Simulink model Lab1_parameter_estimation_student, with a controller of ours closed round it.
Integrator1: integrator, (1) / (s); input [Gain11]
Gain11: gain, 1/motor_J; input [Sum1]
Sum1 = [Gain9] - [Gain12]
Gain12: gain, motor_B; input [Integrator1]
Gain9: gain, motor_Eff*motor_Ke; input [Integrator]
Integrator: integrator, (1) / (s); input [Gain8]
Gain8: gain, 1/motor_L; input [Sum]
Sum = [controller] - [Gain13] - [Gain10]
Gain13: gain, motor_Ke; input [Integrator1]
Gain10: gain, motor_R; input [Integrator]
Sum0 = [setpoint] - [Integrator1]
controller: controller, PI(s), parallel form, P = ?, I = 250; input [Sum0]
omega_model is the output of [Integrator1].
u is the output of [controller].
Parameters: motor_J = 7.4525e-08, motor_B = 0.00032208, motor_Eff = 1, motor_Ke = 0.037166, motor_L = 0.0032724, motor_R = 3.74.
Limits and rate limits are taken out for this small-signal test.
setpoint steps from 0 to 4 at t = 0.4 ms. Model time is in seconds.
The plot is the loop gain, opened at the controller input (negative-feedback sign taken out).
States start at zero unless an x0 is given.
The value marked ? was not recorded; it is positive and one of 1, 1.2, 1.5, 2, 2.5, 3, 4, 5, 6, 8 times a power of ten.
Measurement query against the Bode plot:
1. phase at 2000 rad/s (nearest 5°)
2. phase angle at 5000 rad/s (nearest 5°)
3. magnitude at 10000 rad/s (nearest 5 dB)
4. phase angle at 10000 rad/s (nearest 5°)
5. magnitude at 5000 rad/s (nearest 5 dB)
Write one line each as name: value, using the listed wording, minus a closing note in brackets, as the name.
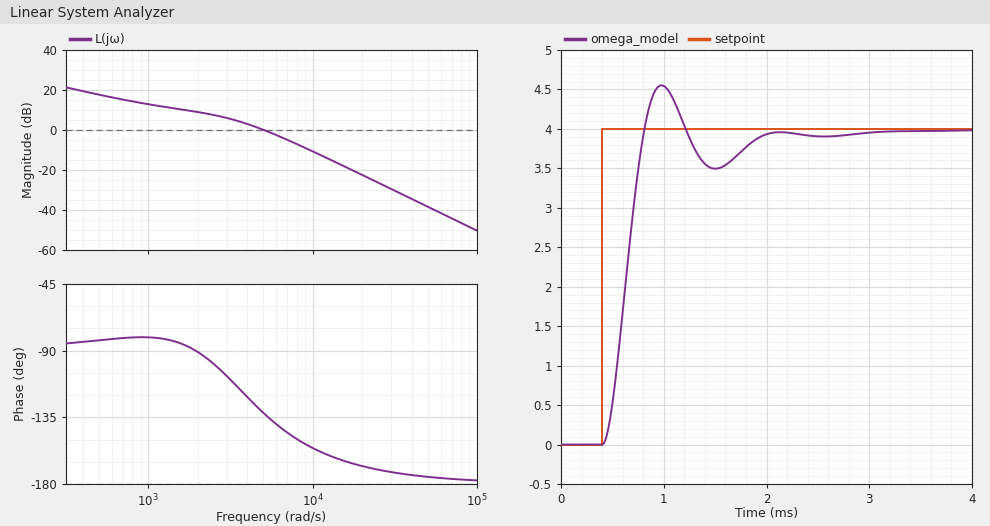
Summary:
phase at 2000 rad/s: -90°
phase angle at 5000 rad/s: -130°
magnitude at 10000 rad/s: -10 dB
phase angle at 10000 rad/s: -155°
magnitude at 5000 rad/s: 0 dB
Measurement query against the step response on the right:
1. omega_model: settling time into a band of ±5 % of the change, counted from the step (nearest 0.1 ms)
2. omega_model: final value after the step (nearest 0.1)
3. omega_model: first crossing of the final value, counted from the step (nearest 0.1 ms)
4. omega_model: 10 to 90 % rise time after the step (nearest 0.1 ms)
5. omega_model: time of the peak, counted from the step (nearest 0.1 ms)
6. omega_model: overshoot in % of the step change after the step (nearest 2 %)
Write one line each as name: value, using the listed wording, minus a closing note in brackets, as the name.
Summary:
omega_model: settling time into a band of ±5 % of the change, counted from the step: 1.4 ms
omega_model: final value after the step: 4.0
omega_model: first crossing of the final value, counted from the step: 0.4 ms
omega_model: 10 to 90 % rise time after the step: 0.3 ms
omega_model: time of the peak, counted from the step: 0.6 ms
omega_model: overshoot in % of the step change after the step: 14 %
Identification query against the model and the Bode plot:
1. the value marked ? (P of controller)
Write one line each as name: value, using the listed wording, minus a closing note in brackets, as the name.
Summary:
the value marked ?: 0.2
